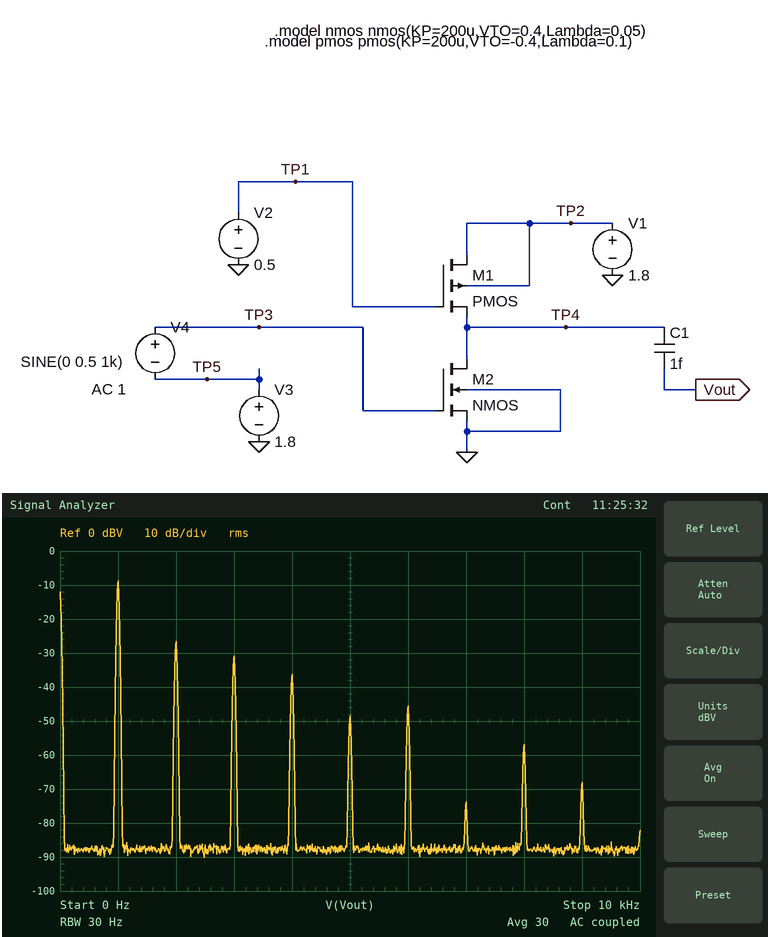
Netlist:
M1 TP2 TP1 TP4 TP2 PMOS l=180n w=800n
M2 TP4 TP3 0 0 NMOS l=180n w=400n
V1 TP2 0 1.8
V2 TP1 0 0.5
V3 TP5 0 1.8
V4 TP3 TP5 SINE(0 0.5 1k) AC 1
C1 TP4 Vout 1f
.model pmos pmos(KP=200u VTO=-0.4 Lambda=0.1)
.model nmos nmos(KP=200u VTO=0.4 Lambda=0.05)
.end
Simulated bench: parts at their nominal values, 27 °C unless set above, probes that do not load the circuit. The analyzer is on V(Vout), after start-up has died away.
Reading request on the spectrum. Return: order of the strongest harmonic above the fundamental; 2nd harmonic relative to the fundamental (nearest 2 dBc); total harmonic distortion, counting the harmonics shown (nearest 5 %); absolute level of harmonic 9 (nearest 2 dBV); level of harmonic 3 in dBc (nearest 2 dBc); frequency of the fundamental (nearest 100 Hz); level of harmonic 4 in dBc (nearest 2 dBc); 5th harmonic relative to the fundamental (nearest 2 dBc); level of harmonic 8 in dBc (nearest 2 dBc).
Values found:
2
-18 dBc
15 %
-68 dBV
-22 dBc
1.0 kHz
-28 dBc
-40 dBc
-48 dBc
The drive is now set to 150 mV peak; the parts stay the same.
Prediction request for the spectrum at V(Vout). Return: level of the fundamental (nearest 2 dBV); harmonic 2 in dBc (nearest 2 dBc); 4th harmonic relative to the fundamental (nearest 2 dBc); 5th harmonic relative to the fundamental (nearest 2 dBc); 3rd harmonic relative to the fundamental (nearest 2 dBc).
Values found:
-18 dBV
-20 dBc
-44 dBc
-50 dBc
-38 dBc
